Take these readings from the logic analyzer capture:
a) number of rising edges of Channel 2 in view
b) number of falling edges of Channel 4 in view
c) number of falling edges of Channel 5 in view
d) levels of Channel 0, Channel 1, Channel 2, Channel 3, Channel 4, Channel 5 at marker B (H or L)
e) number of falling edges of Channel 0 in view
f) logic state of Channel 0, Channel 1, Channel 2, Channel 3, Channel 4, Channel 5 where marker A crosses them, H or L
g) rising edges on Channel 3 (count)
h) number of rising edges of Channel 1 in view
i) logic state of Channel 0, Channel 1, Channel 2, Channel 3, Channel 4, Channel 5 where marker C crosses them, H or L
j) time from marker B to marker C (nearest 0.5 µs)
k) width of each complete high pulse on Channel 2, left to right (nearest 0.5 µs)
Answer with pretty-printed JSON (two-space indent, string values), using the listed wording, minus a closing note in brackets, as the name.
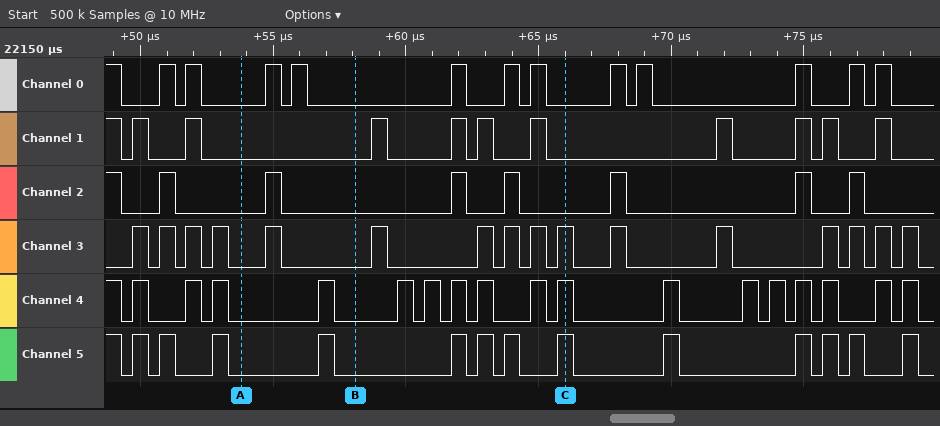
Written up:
{
  "number of rising edges of Channel 2 in view": "7",
  "number of falling edges of Channel 4 in view": "18",
  "number of falling edges of Channel 5 in view": "14",
  "levels of Channel 0, Channel 1, Channel 2, Channel 3, Channel 4, Channel 5 at marker B": "Channel 0=L, Channel 1=L, Channel 2=L, Channel 3=L, Channel 4=L, Channel 5=L",
  "number of falling edges of Channel 0 in view": "13",
  "logic state of Channel 0, Channel 1, Channel 2, Channel 3, Channel 4, Channel 5 where marker A crosses them, H or L": "Channel 0=L, Channel 1=L, Channel 2=L, Channel 3=L, Channel 4=L, Channel 5=L",
  "rising edges on Channel 3": "16",
  "number of rising edges of Channel 1 in view": "10",
  "logic state of Channel 0, Channel 1, Channel 2, Channel 3, Channel 4, Channel 5 where marker C crosses them, H or L": "Channel 0=L, Channel 1=L, Channel 2=L, Channel 3=H, Channel 4=H, Channel 5=H",
  "time from marker B to marker C": "8 µs",
  "width of each complete high pulse on Channel 2, left to right": "0.5 µs, 0.5 µs, 0.5 µs, 0.5 µs, 0.5 µs, 0.5 µs, 0.5 µs"
}
